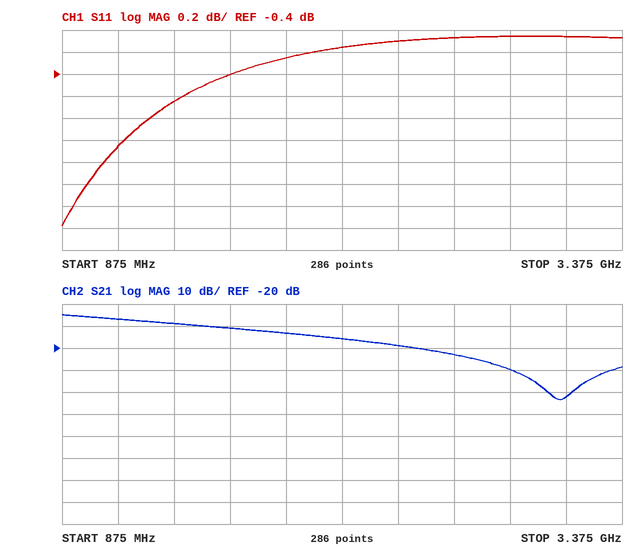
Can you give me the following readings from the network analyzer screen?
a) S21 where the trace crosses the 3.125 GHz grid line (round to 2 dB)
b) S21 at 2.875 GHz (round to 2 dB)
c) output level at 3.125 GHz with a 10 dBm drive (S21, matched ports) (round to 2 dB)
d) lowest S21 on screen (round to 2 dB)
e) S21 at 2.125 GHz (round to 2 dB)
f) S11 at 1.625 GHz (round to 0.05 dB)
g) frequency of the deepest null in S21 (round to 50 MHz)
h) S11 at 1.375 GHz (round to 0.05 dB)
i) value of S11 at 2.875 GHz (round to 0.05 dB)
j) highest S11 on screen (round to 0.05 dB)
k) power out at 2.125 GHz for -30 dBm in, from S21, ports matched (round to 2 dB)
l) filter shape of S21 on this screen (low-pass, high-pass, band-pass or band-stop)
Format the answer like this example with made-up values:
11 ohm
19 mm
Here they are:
-42 dB
-30 dB
-32 dBm
-44 dB
-16 dB
-0.40 dB
3.10 GHz
-0.65 dB
-0.05 dB
-0.05 dB
-46 dBm
low-pass
